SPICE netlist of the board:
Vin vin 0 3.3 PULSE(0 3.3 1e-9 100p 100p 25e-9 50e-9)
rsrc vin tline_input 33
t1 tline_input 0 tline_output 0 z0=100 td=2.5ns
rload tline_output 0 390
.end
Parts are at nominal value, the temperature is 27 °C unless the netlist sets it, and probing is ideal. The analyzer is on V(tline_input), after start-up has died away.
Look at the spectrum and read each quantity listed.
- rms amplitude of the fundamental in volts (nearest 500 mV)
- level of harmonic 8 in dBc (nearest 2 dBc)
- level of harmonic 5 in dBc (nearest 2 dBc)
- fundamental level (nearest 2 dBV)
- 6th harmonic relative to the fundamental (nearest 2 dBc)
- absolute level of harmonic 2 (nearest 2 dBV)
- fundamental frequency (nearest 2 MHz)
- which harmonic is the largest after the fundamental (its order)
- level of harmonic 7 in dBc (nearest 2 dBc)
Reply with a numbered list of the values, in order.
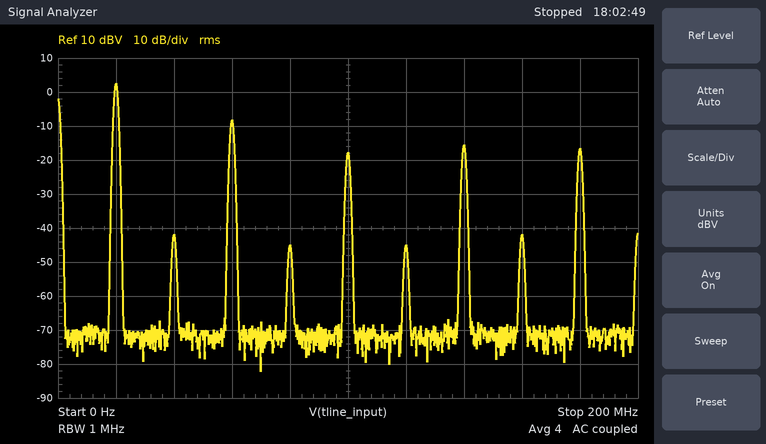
1. 1.5 V
2. -44 dBc
3. -20 dBc
4. 2 dBV
5. -48 dBc
6. -42 dBV
7. 20 MHz
8. 3
9. -18 dBc
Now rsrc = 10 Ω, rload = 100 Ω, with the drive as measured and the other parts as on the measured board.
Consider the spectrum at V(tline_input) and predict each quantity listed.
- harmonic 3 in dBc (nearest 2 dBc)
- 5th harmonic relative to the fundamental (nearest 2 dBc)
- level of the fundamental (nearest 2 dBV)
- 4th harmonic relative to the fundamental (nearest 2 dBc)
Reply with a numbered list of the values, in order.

1. -10 dBc
2. -14 dBc
3. 2 dBV
4. -44 dBc
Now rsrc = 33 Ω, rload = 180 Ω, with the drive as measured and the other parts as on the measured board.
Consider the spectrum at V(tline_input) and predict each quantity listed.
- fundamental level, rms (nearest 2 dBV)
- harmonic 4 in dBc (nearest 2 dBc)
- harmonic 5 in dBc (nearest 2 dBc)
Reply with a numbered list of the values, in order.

1. 2 dBV
2. -46 dBc
3. -16 dBc
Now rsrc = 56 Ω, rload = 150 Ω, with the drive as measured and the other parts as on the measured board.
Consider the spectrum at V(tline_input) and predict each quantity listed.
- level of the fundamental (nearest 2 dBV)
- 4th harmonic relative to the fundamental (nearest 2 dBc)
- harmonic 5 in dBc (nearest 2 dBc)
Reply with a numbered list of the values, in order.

1. 0 dBV
2. -46 dBc
3. -16 dBc
